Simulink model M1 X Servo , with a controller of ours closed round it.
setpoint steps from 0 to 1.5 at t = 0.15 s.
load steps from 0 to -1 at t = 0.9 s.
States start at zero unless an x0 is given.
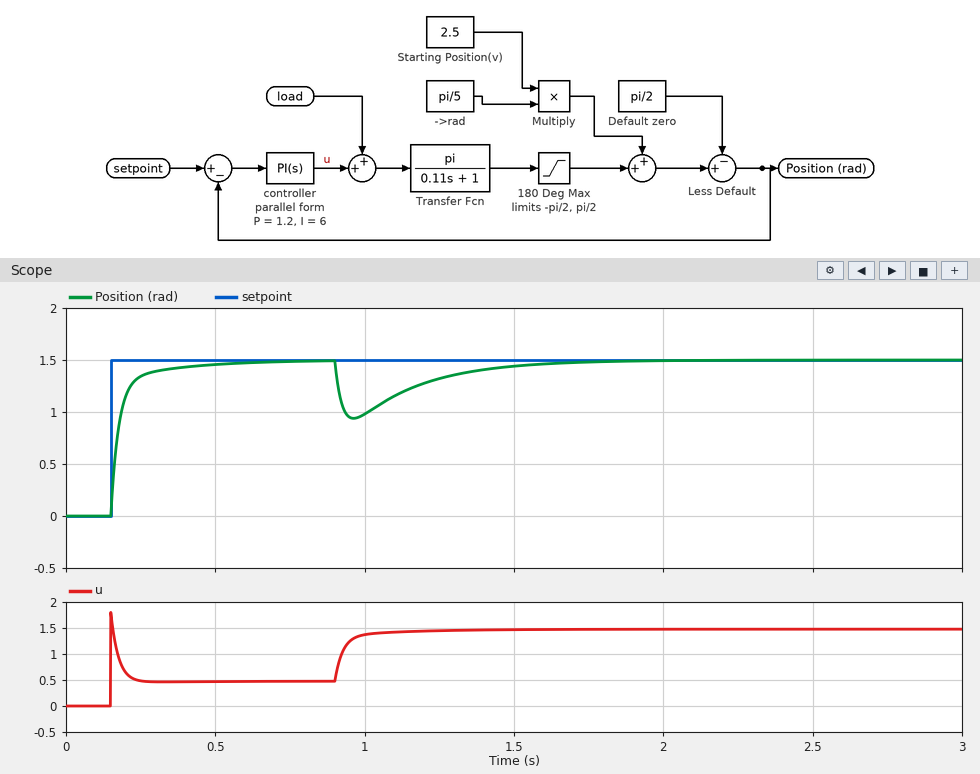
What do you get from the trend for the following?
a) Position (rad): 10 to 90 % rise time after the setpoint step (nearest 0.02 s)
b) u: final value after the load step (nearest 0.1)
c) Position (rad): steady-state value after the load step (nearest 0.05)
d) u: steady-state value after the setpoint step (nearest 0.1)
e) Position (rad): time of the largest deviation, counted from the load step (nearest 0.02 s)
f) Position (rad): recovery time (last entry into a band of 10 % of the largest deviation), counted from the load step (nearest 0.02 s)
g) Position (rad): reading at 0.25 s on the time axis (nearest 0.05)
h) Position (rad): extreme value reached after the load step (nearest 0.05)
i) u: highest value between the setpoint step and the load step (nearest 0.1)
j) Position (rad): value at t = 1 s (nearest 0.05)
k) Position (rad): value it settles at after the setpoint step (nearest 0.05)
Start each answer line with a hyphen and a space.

- 0.10 s
- 1.5
- 1.50
- 0.5
- 0.06 s
- 0.62 s
- 1.35
- 0.95
- 1.8
- 1.00
- 1.50
